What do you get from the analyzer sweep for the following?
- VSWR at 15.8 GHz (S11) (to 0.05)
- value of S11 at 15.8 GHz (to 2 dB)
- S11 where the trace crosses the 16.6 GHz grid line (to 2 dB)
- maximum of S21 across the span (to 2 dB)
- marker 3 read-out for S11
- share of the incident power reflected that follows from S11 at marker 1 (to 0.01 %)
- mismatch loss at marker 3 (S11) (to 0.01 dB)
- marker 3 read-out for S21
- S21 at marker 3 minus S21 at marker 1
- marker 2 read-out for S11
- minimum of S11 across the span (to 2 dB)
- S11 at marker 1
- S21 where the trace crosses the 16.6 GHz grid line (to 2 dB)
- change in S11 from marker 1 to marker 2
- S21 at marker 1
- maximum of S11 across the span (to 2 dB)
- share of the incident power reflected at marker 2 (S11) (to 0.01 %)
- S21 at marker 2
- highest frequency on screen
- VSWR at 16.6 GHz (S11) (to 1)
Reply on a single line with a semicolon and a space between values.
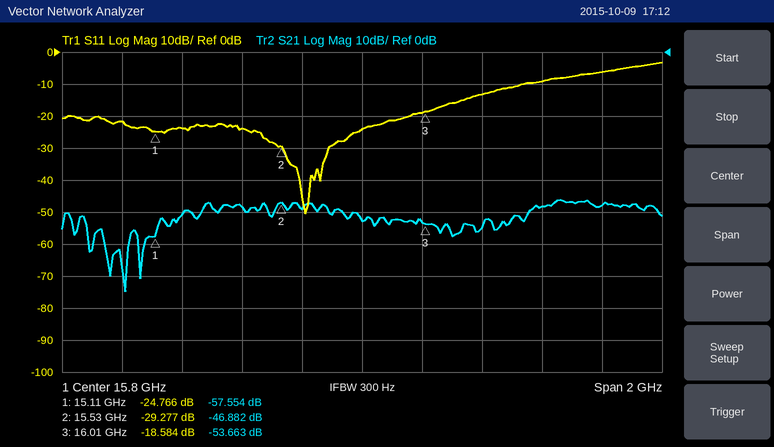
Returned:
1.15; -24 dB; -6 dB; -46 dB; -18.584 dB; 0.33 %; 0.06 dB; -53.663 dB; 3.891 dB; -29.277 dB; -50 dB; -24.766 dB; -48 dB; -4.511 dB; -57.554 dB; -4 dB; 0.12 %; -46.882 dB; 16.8 GHz; 3
